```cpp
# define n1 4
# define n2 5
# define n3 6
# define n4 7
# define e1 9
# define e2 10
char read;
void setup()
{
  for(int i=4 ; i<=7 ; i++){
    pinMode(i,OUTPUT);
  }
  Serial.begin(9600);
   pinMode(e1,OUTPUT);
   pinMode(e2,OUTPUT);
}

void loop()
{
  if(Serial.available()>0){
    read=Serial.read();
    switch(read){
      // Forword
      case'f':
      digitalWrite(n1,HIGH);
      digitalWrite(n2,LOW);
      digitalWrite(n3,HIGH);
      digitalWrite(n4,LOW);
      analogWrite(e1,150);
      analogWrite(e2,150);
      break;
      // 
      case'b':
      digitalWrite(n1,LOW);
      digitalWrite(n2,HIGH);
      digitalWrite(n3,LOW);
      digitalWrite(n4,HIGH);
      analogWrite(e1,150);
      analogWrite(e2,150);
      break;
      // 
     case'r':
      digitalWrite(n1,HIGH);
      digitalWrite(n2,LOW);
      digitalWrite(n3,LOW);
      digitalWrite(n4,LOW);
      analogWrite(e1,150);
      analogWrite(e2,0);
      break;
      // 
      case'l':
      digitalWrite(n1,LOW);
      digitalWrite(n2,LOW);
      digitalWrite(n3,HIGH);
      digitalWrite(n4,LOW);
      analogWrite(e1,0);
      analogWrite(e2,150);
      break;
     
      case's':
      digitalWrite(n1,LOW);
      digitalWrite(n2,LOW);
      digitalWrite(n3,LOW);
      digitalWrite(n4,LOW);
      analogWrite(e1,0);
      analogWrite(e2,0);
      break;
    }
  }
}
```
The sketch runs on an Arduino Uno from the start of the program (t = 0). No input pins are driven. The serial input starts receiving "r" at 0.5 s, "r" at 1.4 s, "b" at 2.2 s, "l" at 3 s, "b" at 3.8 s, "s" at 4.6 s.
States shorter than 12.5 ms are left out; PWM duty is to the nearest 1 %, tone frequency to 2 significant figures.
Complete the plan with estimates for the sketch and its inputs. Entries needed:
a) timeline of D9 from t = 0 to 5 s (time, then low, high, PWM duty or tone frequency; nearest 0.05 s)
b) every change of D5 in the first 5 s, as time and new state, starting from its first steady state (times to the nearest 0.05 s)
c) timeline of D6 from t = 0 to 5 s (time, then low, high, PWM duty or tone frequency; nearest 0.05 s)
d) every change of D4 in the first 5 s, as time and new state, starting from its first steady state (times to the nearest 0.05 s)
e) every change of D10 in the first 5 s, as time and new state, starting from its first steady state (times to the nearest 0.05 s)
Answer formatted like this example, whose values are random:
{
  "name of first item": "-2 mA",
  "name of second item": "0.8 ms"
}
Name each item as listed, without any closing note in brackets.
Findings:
{
  "timeline of D9 from t = 0 to 5 s": "0 s low; 0.5 s PWM 59 %; 3 s low; 3.8 s PWM 59 %; 4.6 s low",
  "every change of D5 in the first 5 s, as time and new state, starting from its first steady state": "0 s low; 2.2 s high; 3 s low; 3.8 s high; 4.6 s low",
  "timeline of D6 from t = 0 to 5 s": "0 s low; 3 s high; 3.8 s low",
  "every change of D4 in the first 5 s, as time and new state, starting from its first steady state": "0 s low; 0.5 s high; 2.2 s low",
  "every change of D10 in the first 5 s, as time and new state, starting from its first steady state": "0 s low; 2.2 s PWM 59 %; 4.6 s low"
}
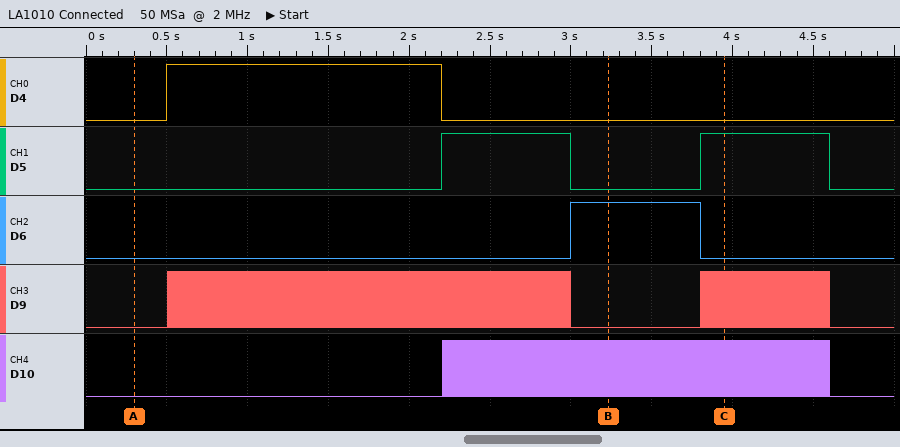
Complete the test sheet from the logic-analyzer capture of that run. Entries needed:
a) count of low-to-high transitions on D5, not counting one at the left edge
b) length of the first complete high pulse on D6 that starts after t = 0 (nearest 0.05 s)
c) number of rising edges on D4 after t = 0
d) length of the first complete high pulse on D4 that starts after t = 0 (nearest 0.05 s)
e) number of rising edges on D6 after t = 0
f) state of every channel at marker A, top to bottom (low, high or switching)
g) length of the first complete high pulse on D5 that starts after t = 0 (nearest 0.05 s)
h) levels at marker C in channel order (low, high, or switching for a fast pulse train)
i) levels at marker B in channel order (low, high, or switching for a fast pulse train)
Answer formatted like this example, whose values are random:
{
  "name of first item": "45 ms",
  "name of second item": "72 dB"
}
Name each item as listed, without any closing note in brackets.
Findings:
{
  "count of low-to-high transitions on D5, not counting one at the left edge": "2",
  "length of the first complete high pulse on D6 that starts after t = 0": "0.80 s",
  "number of rising edges on D4 after t = 0": "1",
  "length of the first complete high pulse on D4 that starts after t = 0": "1.70 s",
  "number of rising edges on D6 after t = 0": "1",
  "state of every channel at marker A, top to bottom": "D4 low, D5 low, D6 low, D9 low, D10 low",
  "length of the first complete high pulse on D5 that starts after t = 0": "0.80 s",
  "levels at marker C in channel order": "D4 low, D5 high, D6 low, D9 switching, D10 switching",
  "levels at marker B in channel order": "D4 low, D5 low, D6 high, D9 low, D10 switching"
}
